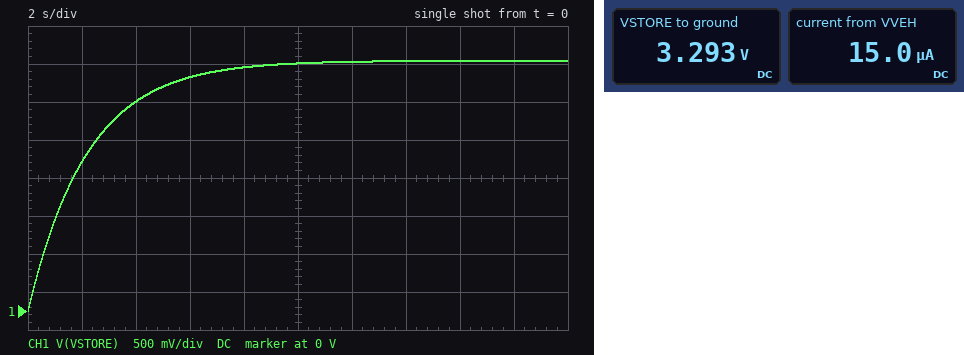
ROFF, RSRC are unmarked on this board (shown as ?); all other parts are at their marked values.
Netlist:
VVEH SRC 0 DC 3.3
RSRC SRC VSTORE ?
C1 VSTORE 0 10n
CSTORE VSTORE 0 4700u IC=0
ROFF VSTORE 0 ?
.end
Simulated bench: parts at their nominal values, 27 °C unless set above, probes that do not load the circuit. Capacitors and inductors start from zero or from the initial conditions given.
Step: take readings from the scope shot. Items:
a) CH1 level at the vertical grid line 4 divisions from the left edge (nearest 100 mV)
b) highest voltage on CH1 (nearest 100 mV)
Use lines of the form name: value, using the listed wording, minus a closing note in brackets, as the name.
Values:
CH1 level at the vertical grid line 4 divisions from the left edge: 3.2 V
highest voltage on CH1: 3.3 V
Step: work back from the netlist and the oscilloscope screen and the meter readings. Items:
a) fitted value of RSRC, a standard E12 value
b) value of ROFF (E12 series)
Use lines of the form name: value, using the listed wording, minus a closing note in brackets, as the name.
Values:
fitted value of RSRC, a standard E12 value: 470 Ω
value of ROFF: 220 kΩ
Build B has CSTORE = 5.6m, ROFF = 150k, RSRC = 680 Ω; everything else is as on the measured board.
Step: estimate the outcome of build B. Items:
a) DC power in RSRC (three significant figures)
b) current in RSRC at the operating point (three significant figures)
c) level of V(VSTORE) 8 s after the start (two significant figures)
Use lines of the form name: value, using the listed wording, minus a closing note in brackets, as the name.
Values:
DC power in RSRC: 326 nW
current in RSRC at the operating point: 21.9 µA
level of V(VSTORE) 8 s after the start: 2.9 V
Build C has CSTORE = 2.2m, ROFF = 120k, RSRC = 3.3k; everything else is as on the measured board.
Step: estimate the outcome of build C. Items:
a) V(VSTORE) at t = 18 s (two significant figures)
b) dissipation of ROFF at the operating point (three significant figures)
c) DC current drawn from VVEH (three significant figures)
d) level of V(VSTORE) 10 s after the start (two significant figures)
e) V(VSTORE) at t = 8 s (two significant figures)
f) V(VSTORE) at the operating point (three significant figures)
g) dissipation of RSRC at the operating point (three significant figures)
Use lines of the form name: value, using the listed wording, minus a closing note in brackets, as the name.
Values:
V(VSTORE) at t = 18 s: 3.0 V
dissipation of ROFF at the operating point: 86.0 µW
DC current drawn from VVEH: 26.8 µA
level of V(VSTORE) 10 s after the start: 2.4 V
V(VSTORE) at t = 8 s: 2.2 V
V(VSTORE) at the operating point: 3.21 V
dissipation of RSRC at the operating point: 2.36 µW
